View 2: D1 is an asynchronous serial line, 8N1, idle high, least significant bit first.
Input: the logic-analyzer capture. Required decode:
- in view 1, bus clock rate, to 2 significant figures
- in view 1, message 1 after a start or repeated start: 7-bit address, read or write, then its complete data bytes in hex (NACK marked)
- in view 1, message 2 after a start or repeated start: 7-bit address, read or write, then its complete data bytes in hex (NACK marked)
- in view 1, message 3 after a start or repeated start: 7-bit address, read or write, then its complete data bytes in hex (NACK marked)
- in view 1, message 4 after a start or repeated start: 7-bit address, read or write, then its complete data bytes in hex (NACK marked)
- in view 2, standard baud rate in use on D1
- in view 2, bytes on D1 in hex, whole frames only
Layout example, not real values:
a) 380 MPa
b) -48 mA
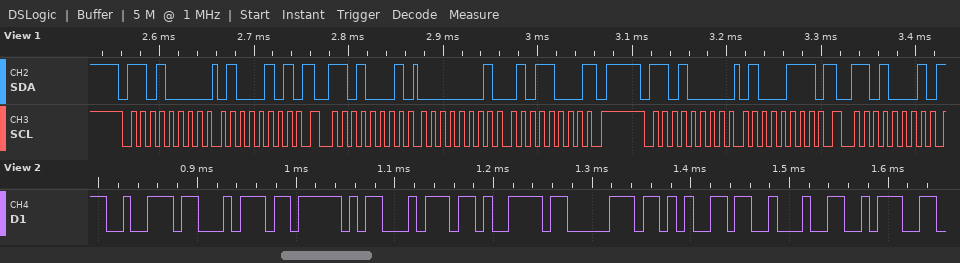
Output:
a) 100 kHz
b) 0x68 write: 45
c) 0x68 read: 01 58 NACK
d) 0x68 write: 47
e) 0x68 read
f) 115200 baud
g) 72 74 5F 74 79 70 65 22 3A
